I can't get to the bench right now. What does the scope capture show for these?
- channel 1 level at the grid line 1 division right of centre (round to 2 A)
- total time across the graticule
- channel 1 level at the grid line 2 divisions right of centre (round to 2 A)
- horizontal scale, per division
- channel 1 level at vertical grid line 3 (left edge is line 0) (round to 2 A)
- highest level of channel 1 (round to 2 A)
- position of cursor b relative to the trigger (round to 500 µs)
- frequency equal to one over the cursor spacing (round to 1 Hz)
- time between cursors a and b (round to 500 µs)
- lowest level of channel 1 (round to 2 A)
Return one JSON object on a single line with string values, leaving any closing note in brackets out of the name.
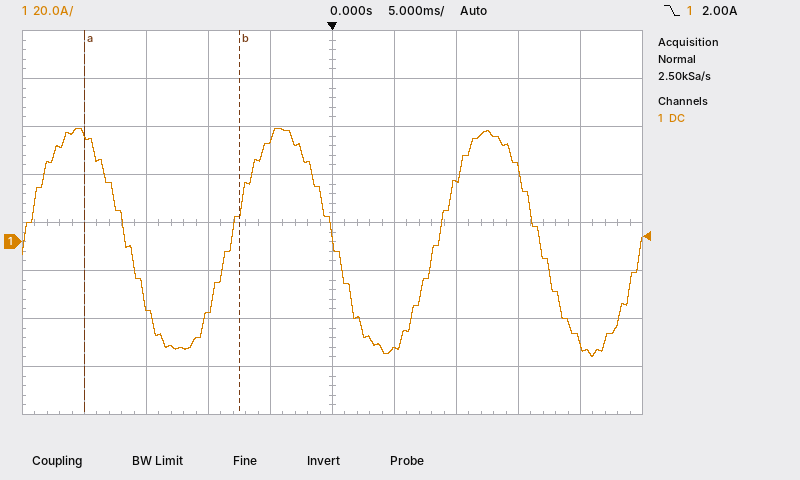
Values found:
{"channel 1 level at the grid line 1 division right of centre": "-44 A", "total time across the graticule": "50 ms", "channel 1 level at the grid line 2 divisions right of centre": "26 A", "horizontal scale, per division": "5 ms", "channel 1 level at vertical grid line 3 (left edge is line 0)": "-28 A", "highest level of channel 1": "48 A", "position of cursor b relative to the trigger": "-7.5 ms", "frequency equal to one over the cursor spacing": "80 Hz", "time between cursors a and b": "12.5 ms", "lowest level of channel 1": "-48 A"}
